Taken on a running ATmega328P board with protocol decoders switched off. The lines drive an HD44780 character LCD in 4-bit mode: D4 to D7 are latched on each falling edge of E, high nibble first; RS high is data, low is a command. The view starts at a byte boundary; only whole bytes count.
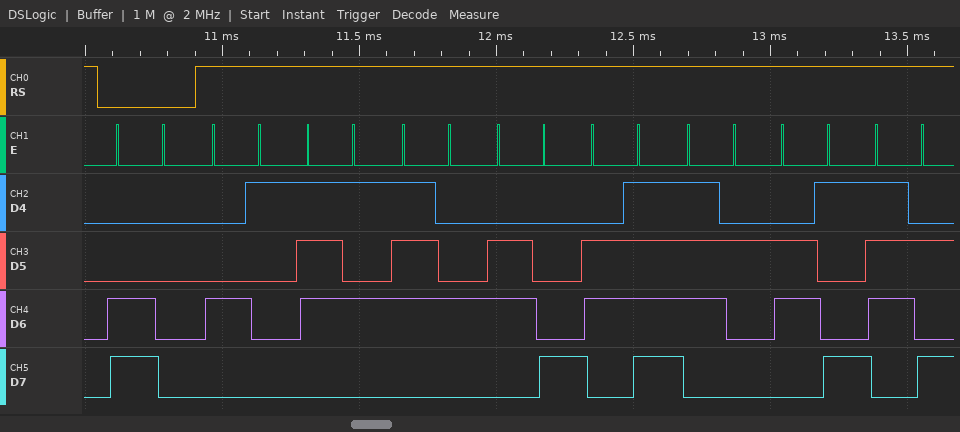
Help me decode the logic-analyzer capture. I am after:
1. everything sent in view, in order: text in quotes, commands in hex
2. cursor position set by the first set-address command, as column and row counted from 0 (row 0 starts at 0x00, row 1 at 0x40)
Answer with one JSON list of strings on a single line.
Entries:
["0xC0 \"Authoriz\"", "column 0, row 1"]
